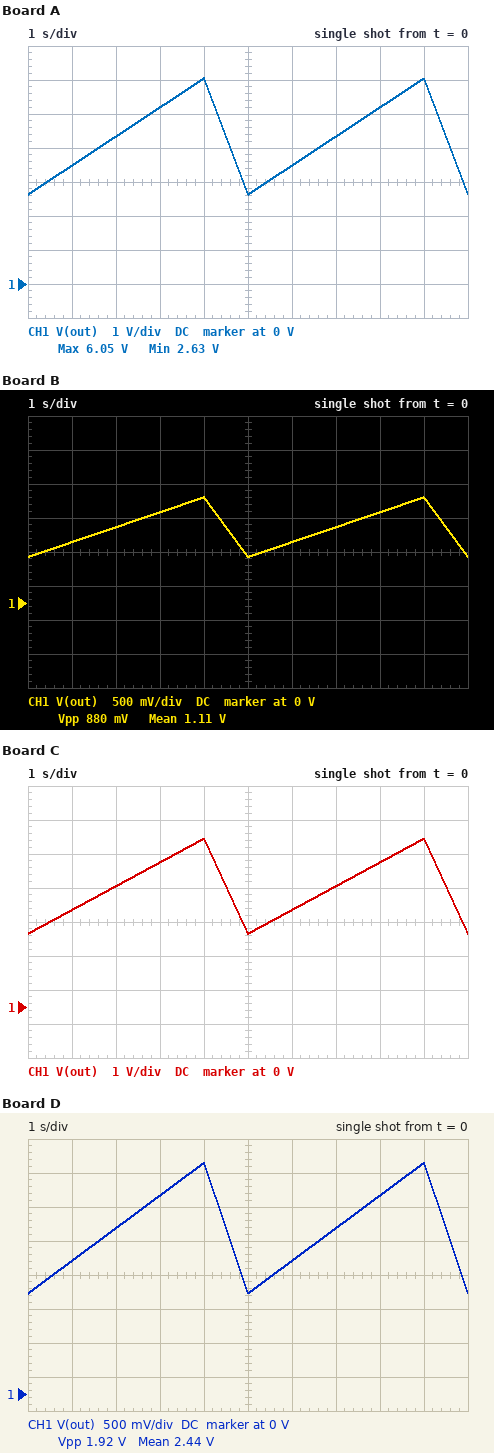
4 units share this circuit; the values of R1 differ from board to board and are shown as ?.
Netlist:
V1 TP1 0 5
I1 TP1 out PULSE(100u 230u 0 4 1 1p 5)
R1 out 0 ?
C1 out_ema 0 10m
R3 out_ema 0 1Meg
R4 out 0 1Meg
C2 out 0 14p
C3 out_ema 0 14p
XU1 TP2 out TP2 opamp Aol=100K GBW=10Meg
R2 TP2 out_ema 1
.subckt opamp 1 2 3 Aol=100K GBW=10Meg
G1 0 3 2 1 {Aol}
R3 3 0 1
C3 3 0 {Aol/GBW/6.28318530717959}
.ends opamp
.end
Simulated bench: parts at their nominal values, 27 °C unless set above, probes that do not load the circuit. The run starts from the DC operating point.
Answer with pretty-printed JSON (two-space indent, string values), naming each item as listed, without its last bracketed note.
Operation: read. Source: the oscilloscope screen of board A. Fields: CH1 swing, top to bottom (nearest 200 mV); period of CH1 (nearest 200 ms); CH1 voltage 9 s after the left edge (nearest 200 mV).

{
  "CH1 swing, top to bottom": "3.4 V",
  "period of CH1": "5.0 s",
  "CH1 voltage 9 s after the left edge": "6.0 V"
}
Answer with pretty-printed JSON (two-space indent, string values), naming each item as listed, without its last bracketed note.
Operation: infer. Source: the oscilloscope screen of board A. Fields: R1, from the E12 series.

{
  "R1, from the E12 series": "27 kΩ"
}
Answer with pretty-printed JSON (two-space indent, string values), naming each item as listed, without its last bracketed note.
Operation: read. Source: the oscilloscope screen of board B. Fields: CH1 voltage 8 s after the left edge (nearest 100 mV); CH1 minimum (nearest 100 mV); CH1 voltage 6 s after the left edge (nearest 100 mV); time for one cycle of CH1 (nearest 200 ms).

{
  "CH1 voltage 8 s after the left edge": "1.3 V",
  "CH1 minimum": "700 mV",
  "CH1 voltage 6 s after the left edge": "900 mV",
  "time for one cycle of CH1": "5.0 s"
}
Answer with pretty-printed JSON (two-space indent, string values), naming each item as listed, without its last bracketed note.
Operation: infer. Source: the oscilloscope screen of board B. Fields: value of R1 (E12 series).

{
  "value of R1": "6.8 kΩ"
}
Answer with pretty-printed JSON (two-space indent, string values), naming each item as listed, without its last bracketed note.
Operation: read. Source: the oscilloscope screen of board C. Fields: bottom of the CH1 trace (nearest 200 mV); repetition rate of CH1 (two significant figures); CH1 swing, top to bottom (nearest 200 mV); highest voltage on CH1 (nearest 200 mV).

{
  "bottom of the CH1 trace": "2.2 V",
  "repetition rate of CH1": "200 mHz",
  "CH1 swing, top to bottom": "2.8 V",
  "highest voltage on CH1": "5.0 V"
}
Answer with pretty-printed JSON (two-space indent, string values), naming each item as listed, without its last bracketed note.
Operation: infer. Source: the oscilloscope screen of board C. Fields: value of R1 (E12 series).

{
  "value of R1": "22 kΩ"
}
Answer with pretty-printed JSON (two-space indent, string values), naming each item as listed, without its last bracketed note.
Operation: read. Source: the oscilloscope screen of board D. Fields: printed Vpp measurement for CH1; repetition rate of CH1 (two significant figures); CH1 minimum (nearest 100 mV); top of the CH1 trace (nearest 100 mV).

{
  "printed Vpp measurement for CH1": "1.92 V",
  "repetition rate of CH1": "200 mHz",
  "CH1 minimum": "1.5 V",
  "top of the CH1 trace": "3.4 V"
}
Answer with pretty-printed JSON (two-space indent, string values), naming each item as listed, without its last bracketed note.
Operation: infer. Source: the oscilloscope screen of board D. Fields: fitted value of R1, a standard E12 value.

{
  "fitted value of R1, a standard E12 value": "15 kΩ"
}
